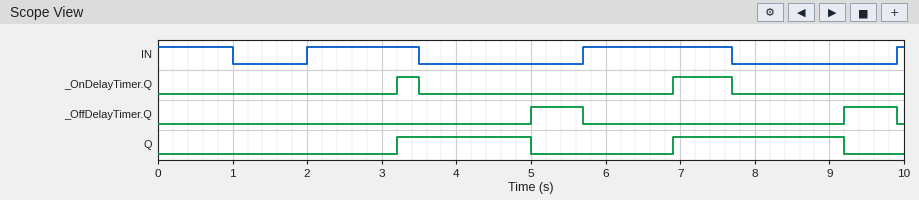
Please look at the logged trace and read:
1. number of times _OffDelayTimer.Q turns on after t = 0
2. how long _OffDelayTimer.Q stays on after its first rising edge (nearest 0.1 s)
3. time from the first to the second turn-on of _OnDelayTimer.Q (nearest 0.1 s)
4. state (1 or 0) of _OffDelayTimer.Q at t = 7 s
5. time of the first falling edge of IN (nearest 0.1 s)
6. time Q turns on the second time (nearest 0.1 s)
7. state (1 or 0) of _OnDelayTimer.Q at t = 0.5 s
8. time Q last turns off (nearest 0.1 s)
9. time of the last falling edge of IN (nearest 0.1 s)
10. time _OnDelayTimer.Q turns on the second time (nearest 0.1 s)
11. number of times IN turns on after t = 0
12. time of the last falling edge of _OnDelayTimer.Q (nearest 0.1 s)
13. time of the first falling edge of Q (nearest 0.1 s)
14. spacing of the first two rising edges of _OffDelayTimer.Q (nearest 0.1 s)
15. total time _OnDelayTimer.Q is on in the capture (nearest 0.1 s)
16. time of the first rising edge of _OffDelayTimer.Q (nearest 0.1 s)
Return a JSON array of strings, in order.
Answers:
["2", "0.7 s", "3.7 s", "0", "1.0 s", "6.9 s", "0", "9.2 s", "7.7 s", "6.9 s", "3", "7.7 s", "5.0 s", "4.2 s", "1.1 s", "5.0 s"]
